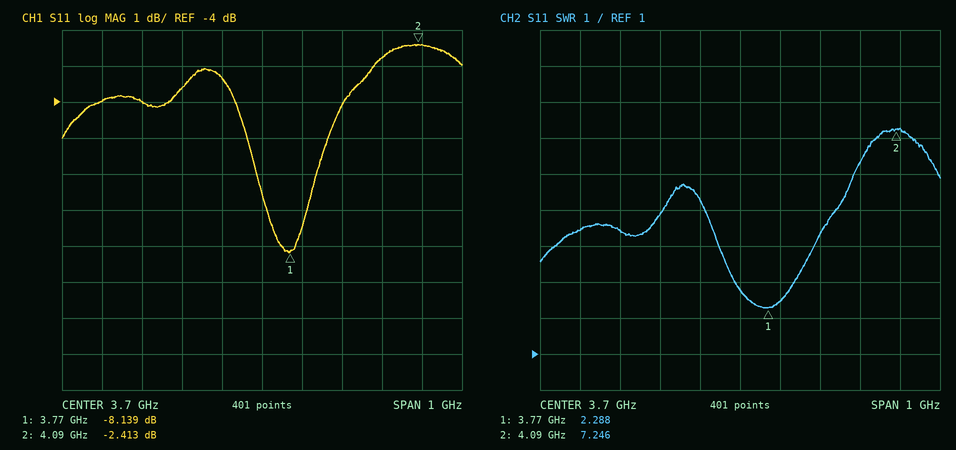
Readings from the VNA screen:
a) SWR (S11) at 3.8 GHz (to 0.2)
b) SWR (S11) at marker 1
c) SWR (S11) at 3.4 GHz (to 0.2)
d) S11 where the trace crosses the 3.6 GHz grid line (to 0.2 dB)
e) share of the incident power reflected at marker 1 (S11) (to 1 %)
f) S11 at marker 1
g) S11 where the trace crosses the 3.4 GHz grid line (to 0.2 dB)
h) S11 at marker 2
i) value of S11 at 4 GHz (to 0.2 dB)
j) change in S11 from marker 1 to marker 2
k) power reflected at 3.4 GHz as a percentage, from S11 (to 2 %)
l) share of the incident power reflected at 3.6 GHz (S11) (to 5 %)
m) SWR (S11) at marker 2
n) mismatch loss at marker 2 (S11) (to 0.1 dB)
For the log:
2.4
2.288
4.4
-3.4 dB
15 %
-8.139 dB
-4.0 dB
-2.413 dB
-2.8 dB
5.726 dB
40 %
45 %
7.246
3.7 dB
